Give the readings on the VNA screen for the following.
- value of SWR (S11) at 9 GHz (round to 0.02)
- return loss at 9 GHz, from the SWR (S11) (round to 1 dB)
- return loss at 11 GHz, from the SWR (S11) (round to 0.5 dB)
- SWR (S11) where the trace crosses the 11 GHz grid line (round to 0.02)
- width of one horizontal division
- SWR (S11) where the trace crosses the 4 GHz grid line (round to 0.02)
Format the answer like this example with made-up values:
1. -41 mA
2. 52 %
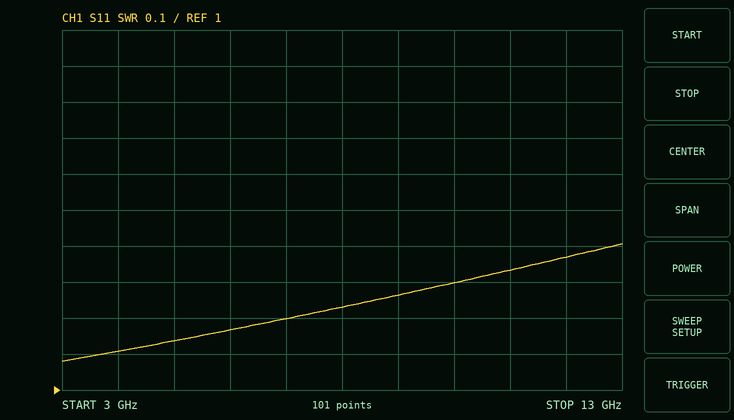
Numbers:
1. 1.26
2. 19 dB
3. 17.0 dB
4. 1.34
5. 1 GHz
6. 1.10
